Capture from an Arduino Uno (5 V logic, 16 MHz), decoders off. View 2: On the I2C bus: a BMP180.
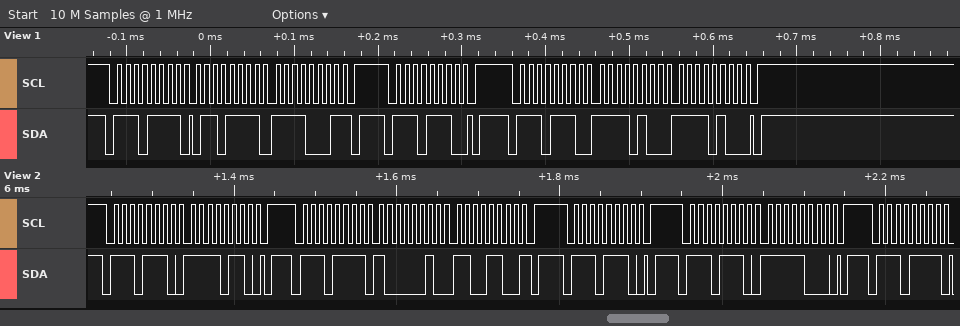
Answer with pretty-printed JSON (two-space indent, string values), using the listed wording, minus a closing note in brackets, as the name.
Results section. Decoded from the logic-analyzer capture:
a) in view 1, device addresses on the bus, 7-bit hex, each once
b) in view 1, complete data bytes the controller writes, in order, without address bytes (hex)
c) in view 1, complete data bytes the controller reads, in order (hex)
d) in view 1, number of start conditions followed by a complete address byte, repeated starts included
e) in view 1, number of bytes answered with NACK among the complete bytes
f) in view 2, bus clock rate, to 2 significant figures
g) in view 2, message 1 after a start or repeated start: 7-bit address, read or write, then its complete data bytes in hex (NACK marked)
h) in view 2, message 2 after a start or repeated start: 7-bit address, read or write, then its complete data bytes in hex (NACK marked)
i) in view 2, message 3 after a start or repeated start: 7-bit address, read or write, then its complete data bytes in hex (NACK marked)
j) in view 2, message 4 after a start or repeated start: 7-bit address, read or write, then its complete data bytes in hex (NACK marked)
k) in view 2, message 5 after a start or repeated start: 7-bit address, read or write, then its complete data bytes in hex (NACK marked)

{
  "in view 1, device addresses on the bus, 7-bit hex, each once": "0x77",
  "in view 1, complete data bytes the controller writes, in order, without address bytes": "F4 F4",
  "in view 1, complete data bytes the controller reads, in order": "6F F1",
  "in view 1, number of start conditions followed by a complete address byte, repeated starts included": "3",
  "in view 1, number of bytes answered with NACK among the complete bytes": "1",
  "in view 2, bus clock rate, to 2 significant figures": "100 kHz",
  "in view 2, message 1 after a start or repeated start: 7-bit address, read or write, then its complete data bytes in hex": "0x77 write: F6",
  "in view 2, message 2 after a start or repeated start: 7-bit address, read or write, then its complete data bytes in hex": "0x77 read: 82 CC NACK",
  "in view 2, message 3 after a start or repeated start: 7-bit address, read or write, then its complete data bytes in hex": "0x77 write",
  "in view 2, message 4 after a start or repeated start: 7-bit address, read or write, then its complete data bytes in hex": "0x77 write: F8",
  "in view 2, message 5 after a start or repeated start: 7-bit address, read or write, then its complete data bytes in hex": "0x77 read"
}
